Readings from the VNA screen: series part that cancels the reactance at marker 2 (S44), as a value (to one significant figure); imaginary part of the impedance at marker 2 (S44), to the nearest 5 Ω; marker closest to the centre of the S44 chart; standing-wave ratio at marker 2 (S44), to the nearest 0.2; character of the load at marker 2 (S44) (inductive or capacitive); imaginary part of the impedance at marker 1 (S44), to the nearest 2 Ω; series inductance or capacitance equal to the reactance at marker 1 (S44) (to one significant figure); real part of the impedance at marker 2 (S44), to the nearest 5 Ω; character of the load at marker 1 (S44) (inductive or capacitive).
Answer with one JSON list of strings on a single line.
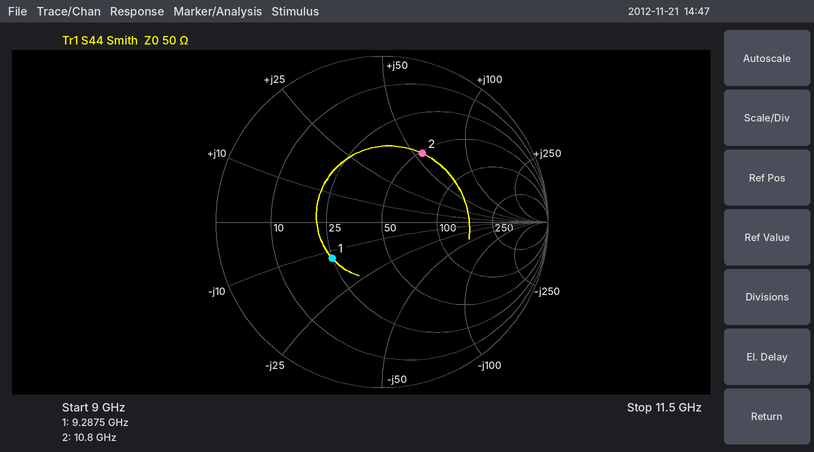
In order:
["300 fF", "+55 Ω", "marker 1", "2.8", "inductive", "-12 Ω", "1 pF", "50 Ω", "capacitive"]
